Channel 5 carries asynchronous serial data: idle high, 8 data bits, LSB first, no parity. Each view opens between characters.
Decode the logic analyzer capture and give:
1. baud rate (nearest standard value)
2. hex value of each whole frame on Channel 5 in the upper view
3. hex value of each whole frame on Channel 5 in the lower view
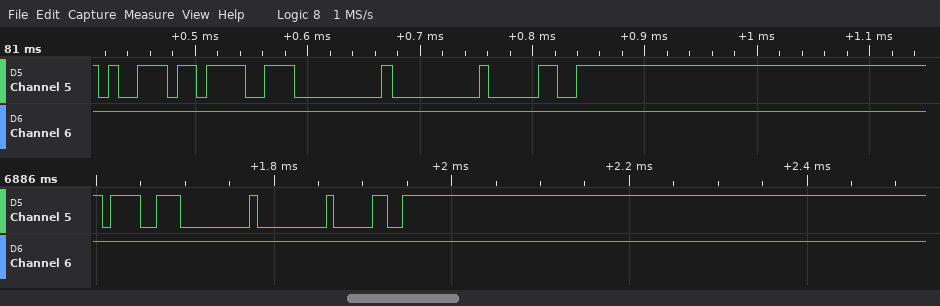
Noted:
115200 baud
B9, CF, 00, 00, 30
CF, 00, 00, 30
